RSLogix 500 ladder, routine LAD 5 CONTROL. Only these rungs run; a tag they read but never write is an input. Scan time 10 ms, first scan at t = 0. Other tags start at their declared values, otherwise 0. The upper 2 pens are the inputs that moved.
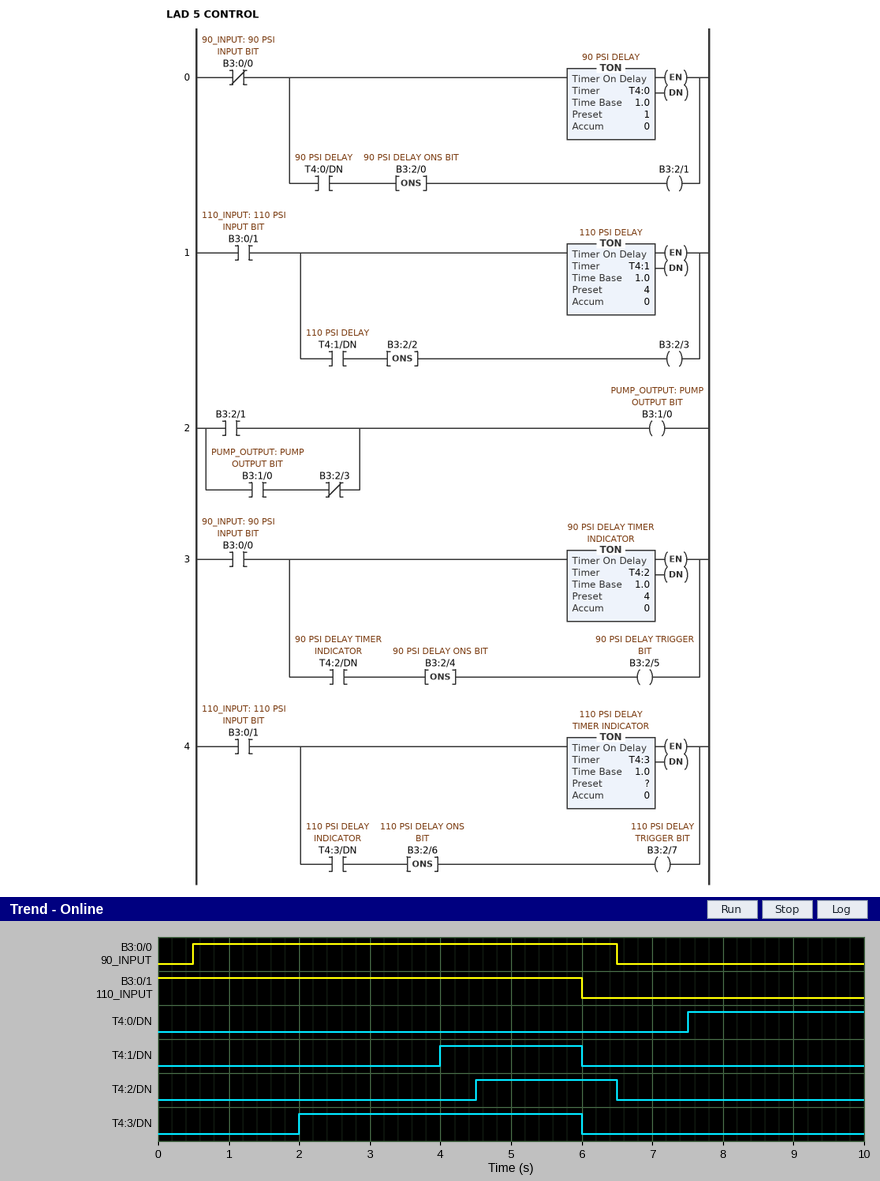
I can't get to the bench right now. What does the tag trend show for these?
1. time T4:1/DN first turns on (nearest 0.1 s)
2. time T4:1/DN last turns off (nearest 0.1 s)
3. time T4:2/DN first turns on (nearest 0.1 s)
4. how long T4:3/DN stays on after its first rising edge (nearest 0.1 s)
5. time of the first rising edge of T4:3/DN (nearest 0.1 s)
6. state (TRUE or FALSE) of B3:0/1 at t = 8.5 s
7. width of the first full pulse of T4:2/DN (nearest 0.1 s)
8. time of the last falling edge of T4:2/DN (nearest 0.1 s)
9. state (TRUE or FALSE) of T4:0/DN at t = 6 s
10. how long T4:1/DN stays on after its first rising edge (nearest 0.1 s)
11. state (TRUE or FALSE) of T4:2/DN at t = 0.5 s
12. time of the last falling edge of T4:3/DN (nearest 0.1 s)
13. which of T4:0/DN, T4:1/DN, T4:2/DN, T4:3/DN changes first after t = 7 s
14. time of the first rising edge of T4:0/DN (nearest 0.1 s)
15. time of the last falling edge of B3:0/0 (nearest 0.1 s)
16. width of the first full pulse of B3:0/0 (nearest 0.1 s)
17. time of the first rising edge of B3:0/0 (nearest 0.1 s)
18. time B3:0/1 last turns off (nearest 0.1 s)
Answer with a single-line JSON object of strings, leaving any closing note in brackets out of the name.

{"time T4:1/DN first turns on": "4.0 s", "time T4:1/DN last turns off": "6.0 s", "time T4:2/DN first turns on": "4.5 s", "how long T4:3/DN stays on after its first rising edge": "4.0 s", "time of the first rising edge of T4:3/DN": "2.0 s", "state (TRUE or FALSE) of B3:0/1 at t = 8.5 s": "FALSE", "width of the first full pulse of T4:2/DN": "2.0 s", "time of the last falling edge of T4:2/DN": "6.5 s", "state (TRUE or FALSE) of T4:0/DN at t = 6 s": "FALSE", "how long T4:1/DN stays on after its first rising edge": "2.0 s", "state (TRUE or FALSE) of T4:2/DN at t = 0.5 s": "FALSE", "time of the last falling edge of T4:3/DN": "6.0 s", "which of T4:0/DN, T4:1/DN, T4:2/DN, T4:3/DN changes first after t = 7 s": "T4:0/DN", "time of the first rising edge of T4:0/DN": "7.5 s", "time of the last falling edge of B3:0/0": "6.5 s", "width of the first full pulse of B3:0/0": "6.0 s", "time of the first rising edge of B3:0/0": "0.5 s", "time B3:0/1 last turns off": "6.0 s"}
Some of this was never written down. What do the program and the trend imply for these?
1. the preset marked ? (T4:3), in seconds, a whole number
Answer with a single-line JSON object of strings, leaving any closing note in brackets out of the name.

{"the preset marked ? (T4:3), in seconds, a whole number": "2 s"}
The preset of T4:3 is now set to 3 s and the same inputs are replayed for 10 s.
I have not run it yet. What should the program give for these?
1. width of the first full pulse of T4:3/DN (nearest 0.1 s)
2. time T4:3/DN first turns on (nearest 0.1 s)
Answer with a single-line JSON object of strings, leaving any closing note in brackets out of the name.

{"width of the first full pulse of T4:3/DN": "3.0 s", "time T4:3/DN first turns on": "3.0 s"}
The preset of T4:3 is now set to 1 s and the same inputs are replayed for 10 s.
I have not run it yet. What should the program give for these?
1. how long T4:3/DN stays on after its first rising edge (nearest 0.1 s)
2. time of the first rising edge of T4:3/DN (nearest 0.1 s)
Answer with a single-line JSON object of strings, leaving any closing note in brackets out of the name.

{"how long T4:3/DN stays on after its first rising edge": "5.0 s", "time of the first rising edge of T4:3/DN": "1.0 s"}
